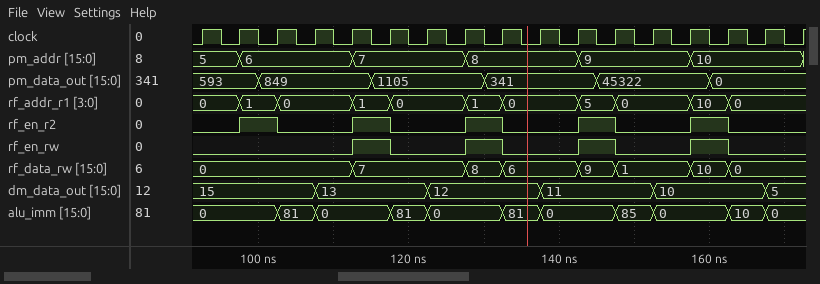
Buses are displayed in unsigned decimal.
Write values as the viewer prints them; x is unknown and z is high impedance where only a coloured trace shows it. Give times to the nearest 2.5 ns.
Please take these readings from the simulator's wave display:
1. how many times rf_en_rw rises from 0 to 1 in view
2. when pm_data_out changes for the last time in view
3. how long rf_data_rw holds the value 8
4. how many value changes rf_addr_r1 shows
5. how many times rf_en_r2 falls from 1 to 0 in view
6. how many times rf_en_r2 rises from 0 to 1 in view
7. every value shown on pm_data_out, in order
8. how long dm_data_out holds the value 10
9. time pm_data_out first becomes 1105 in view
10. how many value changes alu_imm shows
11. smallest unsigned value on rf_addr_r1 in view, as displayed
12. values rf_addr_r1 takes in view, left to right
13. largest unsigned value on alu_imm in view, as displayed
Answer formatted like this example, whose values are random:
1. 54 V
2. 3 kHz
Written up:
1. 4
2. 160 ns
3. 5 ns
4. 10
5. 5
6. 5
7. 593, 849, 1105, 341, 45322, 0
8. 15 ns
9. 115 ns
10. 10
11. 0
12. 0, 1, 0, 1, 0, 1, 0, 5, 0, 10, 0
13. 85
